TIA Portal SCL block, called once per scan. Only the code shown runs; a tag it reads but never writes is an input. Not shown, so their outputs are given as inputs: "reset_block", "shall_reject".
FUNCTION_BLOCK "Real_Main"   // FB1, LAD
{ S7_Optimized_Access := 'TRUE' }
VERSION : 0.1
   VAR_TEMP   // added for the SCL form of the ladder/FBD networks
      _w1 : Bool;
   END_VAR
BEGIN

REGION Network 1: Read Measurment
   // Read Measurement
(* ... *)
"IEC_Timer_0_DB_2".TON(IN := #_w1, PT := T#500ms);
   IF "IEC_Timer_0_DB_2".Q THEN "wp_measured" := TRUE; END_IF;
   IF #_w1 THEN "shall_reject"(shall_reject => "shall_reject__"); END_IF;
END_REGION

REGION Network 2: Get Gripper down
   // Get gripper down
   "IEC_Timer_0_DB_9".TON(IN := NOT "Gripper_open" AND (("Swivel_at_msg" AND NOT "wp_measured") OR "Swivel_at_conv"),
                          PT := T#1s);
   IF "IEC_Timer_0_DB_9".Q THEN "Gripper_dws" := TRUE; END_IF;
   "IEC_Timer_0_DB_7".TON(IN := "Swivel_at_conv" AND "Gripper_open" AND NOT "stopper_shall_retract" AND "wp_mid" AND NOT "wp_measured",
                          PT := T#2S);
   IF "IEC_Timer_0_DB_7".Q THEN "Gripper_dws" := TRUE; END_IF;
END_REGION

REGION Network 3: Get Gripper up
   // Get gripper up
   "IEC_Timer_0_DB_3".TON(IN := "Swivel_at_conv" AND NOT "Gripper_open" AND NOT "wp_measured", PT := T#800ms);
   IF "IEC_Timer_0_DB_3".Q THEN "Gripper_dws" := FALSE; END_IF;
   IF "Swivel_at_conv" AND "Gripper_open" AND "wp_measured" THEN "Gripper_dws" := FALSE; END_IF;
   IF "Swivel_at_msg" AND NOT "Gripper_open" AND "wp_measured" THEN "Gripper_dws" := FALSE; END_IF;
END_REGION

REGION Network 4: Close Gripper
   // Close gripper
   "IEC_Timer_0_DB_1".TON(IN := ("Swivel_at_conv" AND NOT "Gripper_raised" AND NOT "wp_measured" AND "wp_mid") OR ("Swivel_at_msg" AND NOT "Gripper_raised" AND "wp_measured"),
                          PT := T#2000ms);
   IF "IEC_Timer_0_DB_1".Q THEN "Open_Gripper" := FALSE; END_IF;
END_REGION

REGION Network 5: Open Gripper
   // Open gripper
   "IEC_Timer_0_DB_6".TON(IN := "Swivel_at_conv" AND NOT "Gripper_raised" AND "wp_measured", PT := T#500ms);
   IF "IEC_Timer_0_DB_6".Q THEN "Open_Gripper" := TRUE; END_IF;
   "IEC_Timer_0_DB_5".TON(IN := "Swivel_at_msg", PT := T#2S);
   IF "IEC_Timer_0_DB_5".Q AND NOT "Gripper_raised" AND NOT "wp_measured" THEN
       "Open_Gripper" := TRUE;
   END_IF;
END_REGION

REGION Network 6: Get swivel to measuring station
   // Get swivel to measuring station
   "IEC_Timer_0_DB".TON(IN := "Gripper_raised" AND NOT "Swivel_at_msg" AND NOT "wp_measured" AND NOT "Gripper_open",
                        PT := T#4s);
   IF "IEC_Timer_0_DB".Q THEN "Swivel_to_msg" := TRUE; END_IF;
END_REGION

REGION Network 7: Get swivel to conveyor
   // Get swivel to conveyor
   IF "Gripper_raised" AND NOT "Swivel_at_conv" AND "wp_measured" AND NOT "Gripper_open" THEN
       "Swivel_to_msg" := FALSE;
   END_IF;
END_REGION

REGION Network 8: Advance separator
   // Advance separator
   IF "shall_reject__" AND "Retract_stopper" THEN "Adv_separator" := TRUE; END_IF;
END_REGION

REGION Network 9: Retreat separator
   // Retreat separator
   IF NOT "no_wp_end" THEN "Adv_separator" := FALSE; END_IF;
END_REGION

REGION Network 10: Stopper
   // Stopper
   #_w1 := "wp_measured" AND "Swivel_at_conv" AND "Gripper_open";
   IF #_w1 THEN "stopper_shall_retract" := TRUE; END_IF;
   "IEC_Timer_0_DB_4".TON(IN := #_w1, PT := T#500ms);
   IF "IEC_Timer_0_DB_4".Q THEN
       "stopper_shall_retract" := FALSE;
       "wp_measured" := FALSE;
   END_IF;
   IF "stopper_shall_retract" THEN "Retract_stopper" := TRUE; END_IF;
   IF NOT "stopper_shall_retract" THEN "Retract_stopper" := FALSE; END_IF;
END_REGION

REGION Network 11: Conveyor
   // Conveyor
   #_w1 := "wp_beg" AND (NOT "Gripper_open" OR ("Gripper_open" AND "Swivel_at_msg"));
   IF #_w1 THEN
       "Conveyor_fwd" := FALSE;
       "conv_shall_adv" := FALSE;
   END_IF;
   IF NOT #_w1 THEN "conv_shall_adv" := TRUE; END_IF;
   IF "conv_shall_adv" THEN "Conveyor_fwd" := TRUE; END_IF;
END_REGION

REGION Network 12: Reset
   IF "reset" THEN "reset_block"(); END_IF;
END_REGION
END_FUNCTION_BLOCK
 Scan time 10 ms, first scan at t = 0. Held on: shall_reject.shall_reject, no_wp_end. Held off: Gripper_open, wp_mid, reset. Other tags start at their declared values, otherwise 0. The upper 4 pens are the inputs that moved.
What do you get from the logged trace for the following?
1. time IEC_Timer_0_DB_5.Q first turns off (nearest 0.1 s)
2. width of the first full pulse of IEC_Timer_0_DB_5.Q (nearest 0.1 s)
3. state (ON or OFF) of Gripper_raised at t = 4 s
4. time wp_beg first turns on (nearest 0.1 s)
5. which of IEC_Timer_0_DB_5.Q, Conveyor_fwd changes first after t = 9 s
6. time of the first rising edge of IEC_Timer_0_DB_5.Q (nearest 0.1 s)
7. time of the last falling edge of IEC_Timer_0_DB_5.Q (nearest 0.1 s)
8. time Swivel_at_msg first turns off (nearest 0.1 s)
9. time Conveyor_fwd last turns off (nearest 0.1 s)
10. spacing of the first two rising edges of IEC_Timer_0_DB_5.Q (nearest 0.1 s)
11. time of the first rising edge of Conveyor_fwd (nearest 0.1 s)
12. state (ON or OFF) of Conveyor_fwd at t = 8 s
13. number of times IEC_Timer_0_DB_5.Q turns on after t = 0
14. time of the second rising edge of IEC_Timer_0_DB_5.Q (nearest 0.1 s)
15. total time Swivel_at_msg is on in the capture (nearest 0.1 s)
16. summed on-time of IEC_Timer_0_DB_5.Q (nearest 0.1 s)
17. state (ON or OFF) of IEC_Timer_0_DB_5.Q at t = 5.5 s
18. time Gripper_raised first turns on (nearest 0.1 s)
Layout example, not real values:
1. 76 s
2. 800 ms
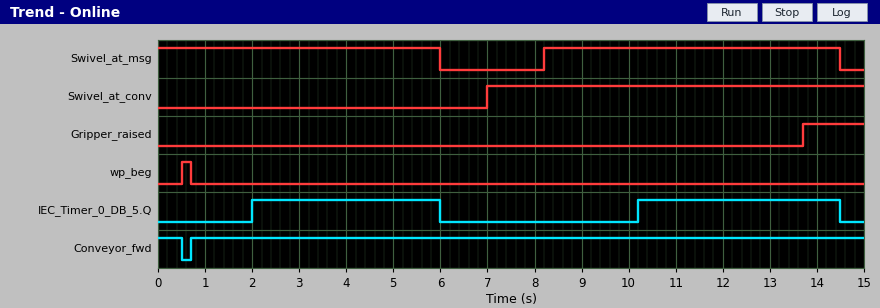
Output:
1. 6.0 s
2. 4.0 s
3. OFF
4. 0.5 s
5. IEC_Timer_0_DB_5.Q
6. 2.0 s
7. 14.5 s
8. 6.0 s
9. 0.5 s
10. 8.2 s
11. 0.7 s
12. ON
13. 2
14. 10.2 s
15. 12.3 s
16. 8.3 s
17. ON
18. 13.7 s
